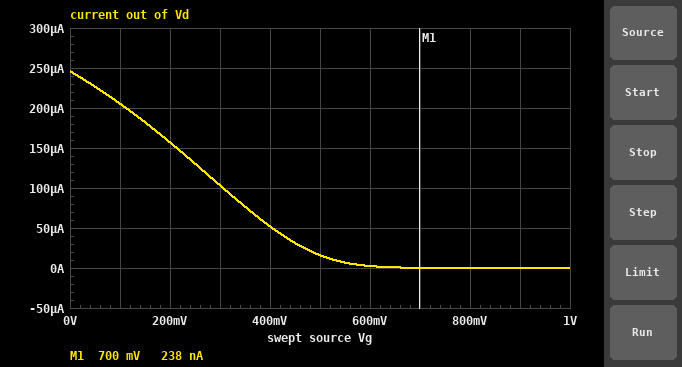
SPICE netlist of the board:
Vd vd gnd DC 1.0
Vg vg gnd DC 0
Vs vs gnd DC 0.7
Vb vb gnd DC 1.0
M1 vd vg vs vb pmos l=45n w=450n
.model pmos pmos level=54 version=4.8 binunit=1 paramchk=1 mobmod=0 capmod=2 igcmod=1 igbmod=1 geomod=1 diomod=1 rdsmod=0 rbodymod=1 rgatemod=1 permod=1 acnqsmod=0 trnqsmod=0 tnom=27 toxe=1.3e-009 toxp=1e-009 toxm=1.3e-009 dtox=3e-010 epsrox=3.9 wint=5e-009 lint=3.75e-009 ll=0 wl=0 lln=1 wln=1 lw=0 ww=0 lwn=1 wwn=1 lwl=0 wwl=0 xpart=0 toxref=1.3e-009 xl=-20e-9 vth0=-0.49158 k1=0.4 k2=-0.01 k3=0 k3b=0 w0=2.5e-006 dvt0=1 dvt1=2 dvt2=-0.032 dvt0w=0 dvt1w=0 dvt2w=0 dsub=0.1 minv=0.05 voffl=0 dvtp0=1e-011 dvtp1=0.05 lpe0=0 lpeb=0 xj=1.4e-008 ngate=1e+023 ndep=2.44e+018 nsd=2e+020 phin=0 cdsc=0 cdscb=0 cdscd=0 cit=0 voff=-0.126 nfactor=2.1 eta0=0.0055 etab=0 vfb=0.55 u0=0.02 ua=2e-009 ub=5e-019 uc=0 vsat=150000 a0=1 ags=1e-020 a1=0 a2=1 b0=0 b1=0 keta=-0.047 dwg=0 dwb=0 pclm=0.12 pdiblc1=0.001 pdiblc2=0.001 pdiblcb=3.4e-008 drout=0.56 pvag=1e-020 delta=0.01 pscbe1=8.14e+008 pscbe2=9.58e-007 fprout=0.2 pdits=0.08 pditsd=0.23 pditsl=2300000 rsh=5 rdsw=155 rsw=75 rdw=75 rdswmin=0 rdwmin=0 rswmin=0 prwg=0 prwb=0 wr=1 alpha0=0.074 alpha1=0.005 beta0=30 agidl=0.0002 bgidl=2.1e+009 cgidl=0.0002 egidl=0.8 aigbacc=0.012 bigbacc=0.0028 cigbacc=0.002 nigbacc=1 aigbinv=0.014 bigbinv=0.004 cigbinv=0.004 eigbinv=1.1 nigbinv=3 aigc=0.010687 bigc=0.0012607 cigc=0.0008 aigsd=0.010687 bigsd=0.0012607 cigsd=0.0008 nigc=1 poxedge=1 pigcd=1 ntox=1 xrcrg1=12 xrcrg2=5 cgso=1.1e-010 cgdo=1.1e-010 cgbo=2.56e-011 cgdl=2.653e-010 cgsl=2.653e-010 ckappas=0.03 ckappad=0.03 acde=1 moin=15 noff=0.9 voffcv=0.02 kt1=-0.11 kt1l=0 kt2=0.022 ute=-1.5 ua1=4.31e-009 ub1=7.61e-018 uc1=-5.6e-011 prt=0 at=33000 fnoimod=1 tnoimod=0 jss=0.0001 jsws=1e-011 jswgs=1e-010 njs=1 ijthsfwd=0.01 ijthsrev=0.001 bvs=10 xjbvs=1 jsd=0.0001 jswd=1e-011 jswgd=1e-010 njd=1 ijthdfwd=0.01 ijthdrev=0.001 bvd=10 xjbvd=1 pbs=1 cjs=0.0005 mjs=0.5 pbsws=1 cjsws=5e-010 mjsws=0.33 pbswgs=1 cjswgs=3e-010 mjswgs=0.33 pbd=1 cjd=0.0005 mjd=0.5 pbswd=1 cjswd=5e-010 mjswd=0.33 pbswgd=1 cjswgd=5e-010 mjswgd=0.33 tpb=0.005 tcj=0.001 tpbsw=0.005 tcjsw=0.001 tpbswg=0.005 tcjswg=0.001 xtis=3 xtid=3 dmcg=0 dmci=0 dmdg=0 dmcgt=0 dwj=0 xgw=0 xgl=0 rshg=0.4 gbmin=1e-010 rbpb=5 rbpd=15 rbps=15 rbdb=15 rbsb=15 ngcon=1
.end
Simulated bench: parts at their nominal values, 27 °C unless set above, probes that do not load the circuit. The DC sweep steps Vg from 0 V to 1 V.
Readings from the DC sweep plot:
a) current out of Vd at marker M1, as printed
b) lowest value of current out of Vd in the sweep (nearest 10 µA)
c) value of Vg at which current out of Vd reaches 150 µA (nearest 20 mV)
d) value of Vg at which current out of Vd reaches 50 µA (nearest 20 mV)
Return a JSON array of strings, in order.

["238 nA", "0 A", "220 mV", "400 mV"]
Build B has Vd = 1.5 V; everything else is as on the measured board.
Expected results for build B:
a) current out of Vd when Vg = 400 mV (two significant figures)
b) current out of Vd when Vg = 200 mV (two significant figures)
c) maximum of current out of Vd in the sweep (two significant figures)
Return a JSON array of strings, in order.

["550 µA", "690 µA", "810 µA"]
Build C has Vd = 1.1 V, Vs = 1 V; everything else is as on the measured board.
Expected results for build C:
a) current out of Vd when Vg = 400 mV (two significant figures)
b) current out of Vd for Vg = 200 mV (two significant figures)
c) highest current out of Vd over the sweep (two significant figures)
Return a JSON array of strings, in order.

["58 µA", "92 µA", "110 µA"]
